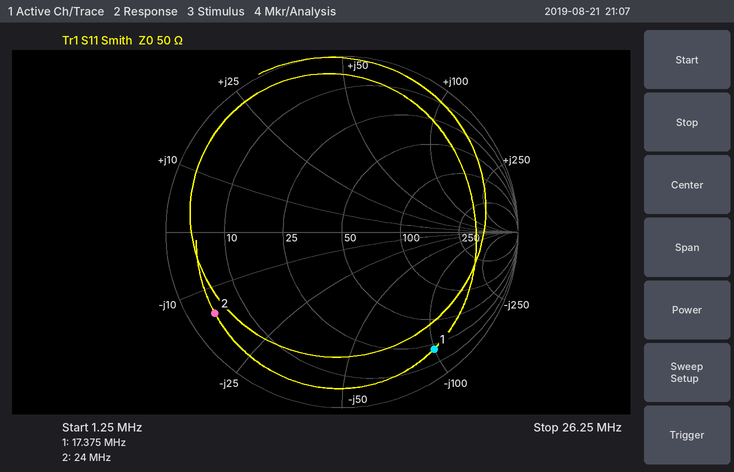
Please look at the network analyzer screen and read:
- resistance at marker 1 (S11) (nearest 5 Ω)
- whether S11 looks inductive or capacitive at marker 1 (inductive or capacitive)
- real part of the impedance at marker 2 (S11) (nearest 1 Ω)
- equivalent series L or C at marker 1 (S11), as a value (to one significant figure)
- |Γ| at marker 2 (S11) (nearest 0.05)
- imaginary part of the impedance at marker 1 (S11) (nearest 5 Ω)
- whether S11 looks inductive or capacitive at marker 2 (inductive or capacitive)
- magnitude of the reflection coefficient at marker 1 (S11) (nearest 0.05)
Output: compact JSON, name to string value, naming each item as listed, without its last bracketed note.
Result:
{"resistance at marker 1 (S11)": "20 Ω", "whether S11 looks inductive or capacitive at marker 1": "capacitive", "real part of the impedance at marker 2 (S11)": "4 Ω", "equivalent series L or C at marker 1 (S11), as a value": "90 pF", "|Γ| at marker 2 (S11)": "0.85", "imaginary part of the impedance at marker 1 (S11)": "-100 Ω", "whether S11 looks inductive or capacitive at marker 2": "capacitive", "magnitude of the reflection coefficient at marker 1 (S11)": "0.85"}
